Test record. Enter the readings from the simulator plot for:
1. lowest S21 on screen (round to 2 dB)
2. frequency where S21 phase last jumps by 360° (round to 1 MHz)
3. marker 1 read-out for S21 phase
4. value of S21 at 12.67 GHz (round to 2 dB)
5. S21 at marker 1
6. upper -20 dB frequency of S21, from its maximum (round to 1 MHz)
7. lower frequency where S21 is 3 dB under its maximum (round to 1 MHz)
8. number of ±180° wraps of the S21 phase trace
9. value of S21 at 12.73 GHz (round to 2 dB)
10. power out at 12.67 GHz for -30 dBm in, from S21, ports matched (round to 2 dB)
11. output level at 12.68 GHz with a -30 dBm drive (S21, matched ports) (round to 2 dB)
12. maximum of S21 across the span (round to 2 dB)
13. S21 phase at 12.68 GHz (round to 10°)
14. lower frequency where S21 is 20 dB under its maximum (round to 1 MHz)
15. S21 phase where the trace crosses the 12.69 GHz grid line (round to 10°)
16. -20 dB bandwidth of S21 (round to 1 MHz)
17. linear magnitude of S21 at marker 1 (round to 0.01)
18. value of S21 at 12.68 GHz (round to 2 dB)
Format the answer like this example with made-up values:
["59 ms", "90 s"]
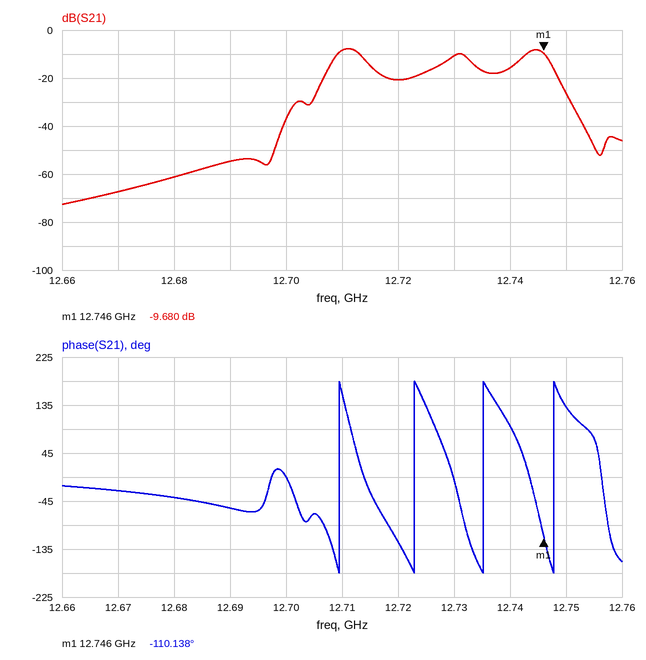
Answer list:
["-72 dB", "12.748 GHz", "-110.138°", "-68 dB", "-9.680 dB", "12.750 GHz", "12.709 GHz", "4", "-10 dB", "-98 dBm", "-92 dBm", "-8 dB", "-40°", "12.705 GHz", "-60°", "45 MHz", "0.33", "-62 dB"]
